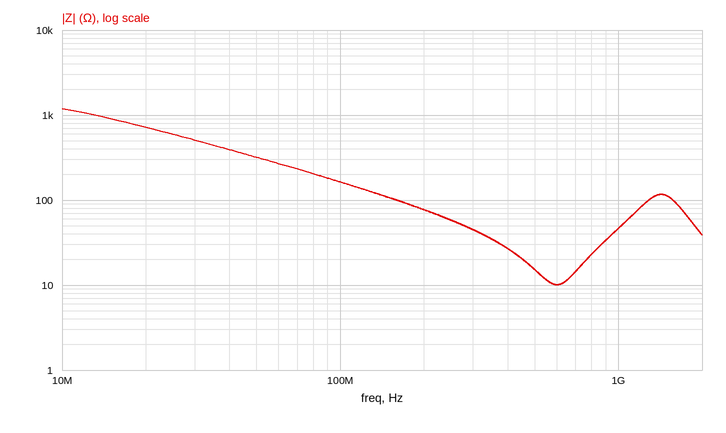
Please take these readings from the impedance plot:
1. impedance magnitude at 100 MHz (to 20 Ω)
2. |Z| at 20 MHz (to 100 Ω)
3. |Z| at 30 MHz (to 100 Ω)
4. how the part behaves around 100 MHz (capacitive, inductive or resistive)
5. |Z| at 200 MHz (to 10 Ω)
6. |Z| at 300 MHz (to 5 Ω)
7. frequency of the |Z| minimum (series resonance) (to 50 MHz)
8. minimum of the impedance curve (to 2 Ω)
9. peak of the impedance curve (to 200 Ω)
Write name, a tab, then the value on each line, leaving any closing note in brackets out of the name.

impedance magnitude at 100 MHz	160 Ω
|Z| at 20 MHz	700 Ω
|Z| at 30 MHz	500 Ω
how the part behaves around 100 MHz	capacitive
|Z| at 200 MHz	80 Ω
|Z| at 300 MHz	45 Ω
frequency of the |Z| minimum (series resonance)	600 MHz
minimum of the impedance curve	10 Ω
peak of the impedance curve	1.2 kΩ
